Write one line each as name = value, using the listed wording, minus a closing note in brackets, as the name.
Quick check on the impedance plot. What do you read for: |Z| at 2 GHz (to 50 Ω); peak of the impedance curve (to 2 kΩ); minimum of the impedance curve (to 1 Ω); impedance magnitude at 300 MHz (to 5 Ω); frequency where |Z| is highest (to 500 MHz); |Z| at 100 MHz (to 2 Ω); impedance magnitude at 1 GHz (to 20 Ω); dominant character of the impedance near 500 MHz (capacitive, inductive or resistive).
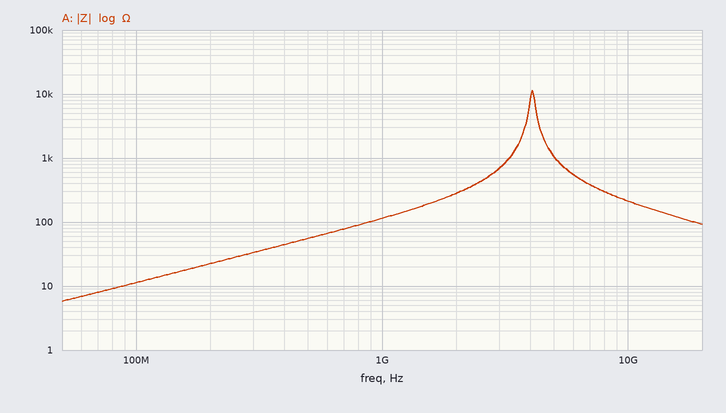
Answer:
|Z| at 2 GHz = 300 Ω
peak of the impedance curve = 12 kΩ
minimum of the impedance curve = 6 Ω
impedance magnitude at 300 MHz = 35 Ω
frequency where |Z| is highest = 4.0 GHz
|Z| at 100 MHz = 12 Ω
impedance magnitude at 1 GHz = 120 Ω
dominant character of the impedance near 500 MHz = inductive
